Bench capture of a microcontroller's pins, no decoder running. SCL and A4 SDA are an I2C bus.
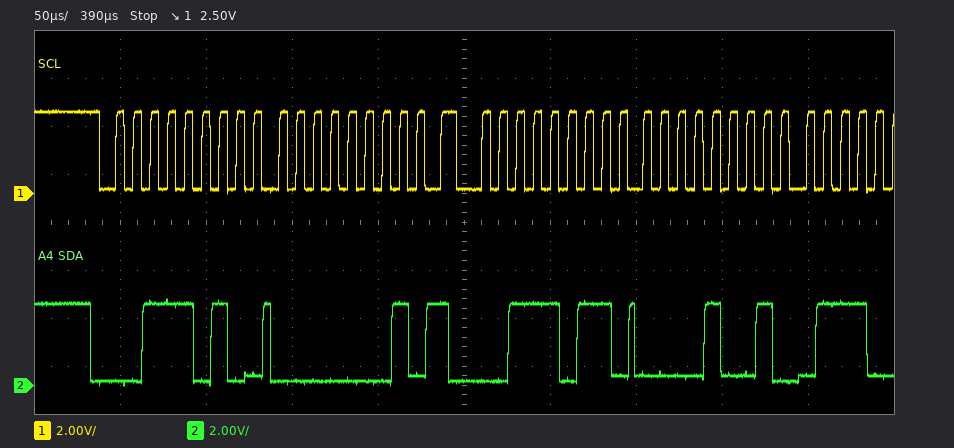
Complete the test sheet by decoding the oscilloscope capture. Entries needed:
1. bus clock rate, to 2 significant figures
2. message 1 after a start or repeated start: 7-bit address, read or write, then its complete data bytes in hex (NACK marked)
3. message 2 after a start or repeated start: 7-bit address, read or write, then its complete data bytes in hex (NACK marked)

100 kHz
0x1D write: 01
0x1D read: 09
